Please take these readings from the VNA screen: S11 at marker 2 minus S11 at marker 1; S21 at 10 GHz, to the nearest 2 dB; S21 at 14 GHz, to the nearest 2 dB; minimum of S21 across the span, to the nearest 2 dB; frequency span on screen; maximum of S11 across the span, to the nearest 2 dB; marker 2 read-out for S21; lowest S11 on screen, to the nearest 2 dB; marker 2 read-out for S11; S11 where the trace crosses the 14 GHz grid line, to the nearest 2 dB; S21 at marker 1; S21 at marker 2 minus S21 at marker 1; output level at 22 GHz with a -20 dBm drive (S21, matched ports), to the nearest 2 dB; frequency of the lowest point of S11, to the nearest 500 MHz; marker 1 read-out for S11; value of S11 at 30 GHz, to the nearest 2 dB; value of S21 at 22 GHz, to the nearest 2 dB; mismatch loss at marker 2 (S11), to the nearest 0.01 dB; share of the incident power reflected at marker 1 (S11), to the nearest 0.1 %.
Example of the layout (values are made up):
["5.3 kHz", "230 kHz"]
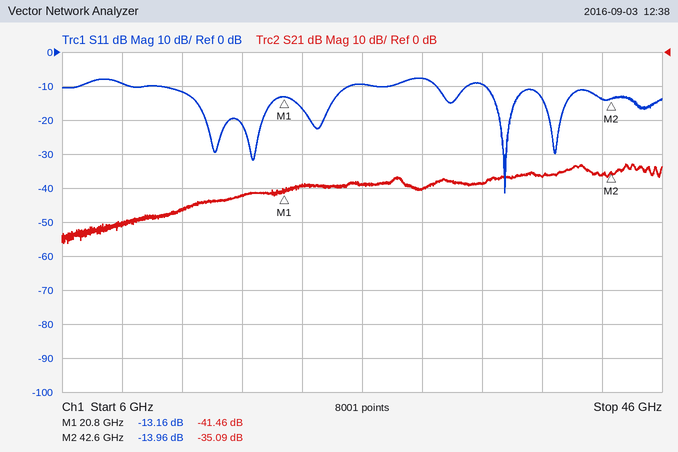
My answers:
["-0.80 dB", "-50 dB", "-46 dB", "-56 dB", "40 GHz", "-8 dB", "-35.09 dB", "-42 dB", "-13.96 dB", "-12 dB", "-41.46 dB", "6.37 dB", "-60 dBm", "35.5 GHz", "-13.16 dB", "-8 dB", "-40 dB", "0.18 dB", "4.8 %"]
